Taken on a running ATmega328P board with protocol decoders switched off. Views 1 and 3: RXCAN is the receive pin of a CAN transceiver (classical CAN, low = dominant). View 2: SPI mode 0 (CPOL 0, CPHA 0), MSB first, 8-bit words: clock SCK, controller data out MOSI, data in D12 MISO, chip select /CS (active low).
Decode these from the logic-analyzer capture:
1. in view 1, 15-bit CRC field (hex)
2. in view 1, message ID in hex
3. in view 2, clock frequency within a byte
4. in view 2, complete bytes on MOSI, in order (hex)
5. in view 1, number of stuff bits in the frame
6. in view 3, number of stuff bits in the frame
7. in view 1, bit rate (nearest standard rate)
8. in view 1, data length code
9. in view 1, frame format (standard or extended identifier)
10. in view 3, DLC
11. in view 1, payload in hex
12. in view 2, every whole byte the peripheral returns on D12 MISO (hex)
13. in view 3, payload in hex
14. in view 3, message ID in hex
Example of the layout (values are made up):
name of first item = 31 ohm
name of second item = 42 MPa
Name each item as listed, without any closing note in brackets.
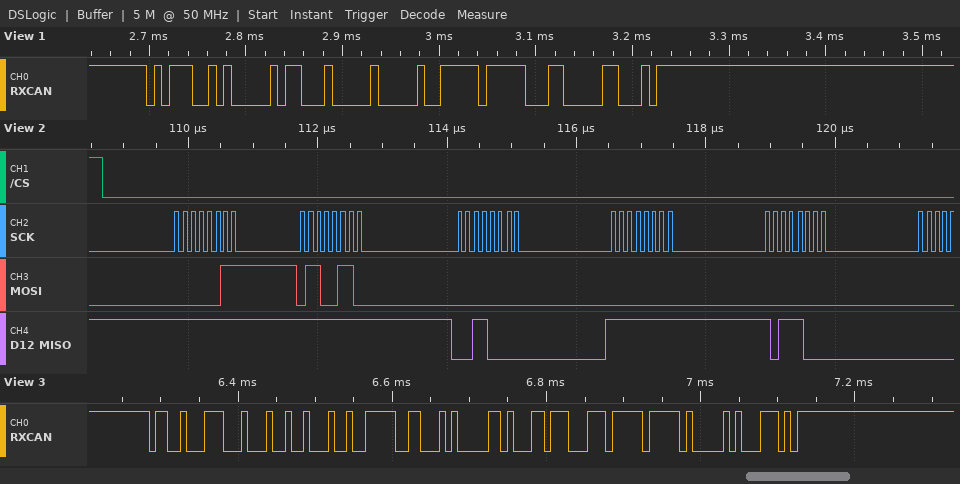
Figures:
in view 1, 15-bit CRC field = 0x6608
in view 1, message ID in hex = 0x5CA
in view 2, clock frequency within a byte = 8 MHz
in view 2, complete bytes on MOSI, in order = 03 66 00 00 00
in view 1, number of stuff bits in the frame = 6
in view 3, number of stuff bits in the frame = 5
in view 1, bit rate = 125 kbit/s
in view 1, data length code = 3
in view 1, frame format = standard
in view 3, DLC = 8
in view 1, payload in hex = 10 00 FF
in view 2, every whole byte the peripheral returns on D12 MISO = FF FF 30 FF B8
in view 3, payload in hex = 92 24 FB 14 14 6E 3B FF
in view 3, message ID in hex = 0x647
